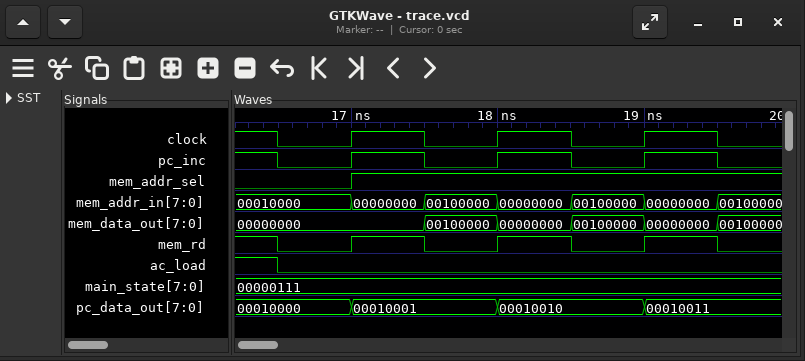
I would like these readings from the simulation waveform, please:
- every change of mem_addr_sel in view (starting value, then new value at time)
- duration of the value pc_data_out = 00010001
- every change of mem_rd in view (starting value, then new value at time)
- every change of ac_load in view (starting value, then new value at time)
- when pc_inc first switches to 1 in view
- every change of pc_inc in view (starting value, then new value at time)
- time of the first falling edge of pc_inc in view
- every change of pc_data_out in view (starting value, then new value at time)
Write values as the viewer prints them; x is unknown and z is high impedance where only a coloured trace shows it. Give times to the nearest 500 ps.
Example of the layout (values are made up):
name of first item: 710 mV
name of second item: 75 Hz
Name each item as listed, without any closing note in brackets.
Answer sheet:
every change of mem_addr_sel in view: 0, 1 at 17000 ps
duration of the value pc_data_out = 00010001: 1000 ps
every change of mem_rd in view: 1, 0 at 16500 ps, 1 at 17000 ps, 0 at 17500 ps, 1 at 18000 ps, 0 at 18500 ps, 1 at 19000 ps, 0 at 19500 ps
every change of ac_load in view: 1, 0 at 16500 ps
when pc_inc first switches to 1 in view: 17000 ps
every change of pc_inc in view: 1, 0 at 16500 ps, 1 at 17000 ps, 0 at 17500 ps, 1 at 18000 ps, 0 at 18500 ps, 1 at 19000 ps, 0 at 19500 ps
time of the first falling edge of pc_inc in view: 16500 ps
every change of pc_data_out in view: 00010000, 00010001 at 17000 ps, 00010010 at 18000 ps, 00010011 at 19000 ps
